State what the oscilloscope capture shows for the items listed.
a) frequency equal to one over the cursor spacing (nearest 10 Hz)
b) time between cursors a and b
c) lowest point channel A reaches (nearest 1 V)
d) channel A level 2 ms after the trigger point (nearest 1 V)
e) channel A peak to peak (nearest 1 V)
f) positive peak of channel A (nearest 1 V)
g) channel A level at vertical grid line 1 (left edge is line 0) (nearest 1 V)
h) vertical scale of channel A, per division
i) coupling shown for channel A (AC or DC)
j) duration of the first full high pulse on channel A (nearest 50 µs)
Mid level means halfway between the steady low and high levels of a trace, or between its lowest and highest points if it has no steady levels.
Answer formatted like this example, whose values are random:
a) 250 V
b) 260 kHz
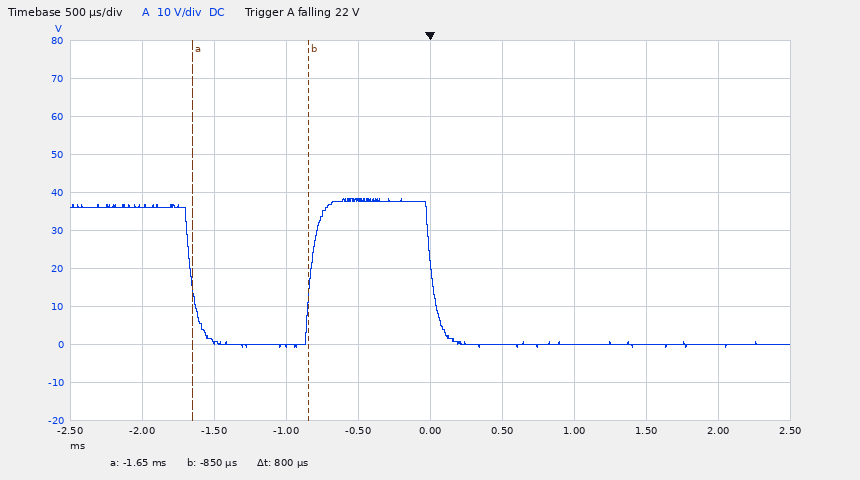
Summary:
a) 1.25 kHz
b) 800 µs
c) -1 V
d) 0 V
e) 39 V
f) 38 V
g) 36 V
h) 10 V
i) DC
j) 850 µs
